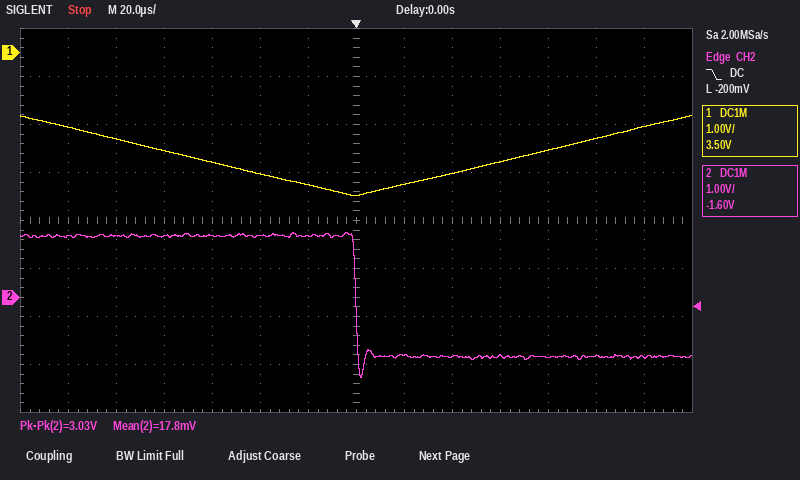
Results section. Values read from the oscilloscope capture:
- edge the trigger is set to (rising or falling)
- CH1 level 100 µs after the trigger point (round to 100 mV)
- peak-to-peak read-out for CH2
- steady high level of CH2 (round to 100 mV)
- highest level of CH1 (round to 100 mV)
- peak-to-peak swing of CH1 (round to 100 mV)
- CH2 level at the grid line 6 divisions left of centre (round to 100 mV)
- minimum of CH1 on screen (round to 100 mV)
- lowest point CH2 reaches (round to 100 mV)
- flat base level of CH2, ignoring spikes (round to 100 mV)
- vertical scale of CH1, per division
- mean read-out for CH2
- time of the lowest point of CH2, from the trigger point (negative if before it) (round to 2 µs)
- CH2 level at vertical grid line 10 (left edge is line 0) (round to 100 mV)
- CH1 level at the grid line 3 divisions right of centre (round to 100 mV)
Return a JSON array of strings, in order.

["falling", "-1.8 V", "3.03 V", "1.3 V", "-1.3 V", "1.7 V", "1.3 V", "-3.0 V", "-1.7 V", "-1.2 V", "1 V", "17.8 mV", "+2 µs", "-1.2 V", "-2.3 V"]
